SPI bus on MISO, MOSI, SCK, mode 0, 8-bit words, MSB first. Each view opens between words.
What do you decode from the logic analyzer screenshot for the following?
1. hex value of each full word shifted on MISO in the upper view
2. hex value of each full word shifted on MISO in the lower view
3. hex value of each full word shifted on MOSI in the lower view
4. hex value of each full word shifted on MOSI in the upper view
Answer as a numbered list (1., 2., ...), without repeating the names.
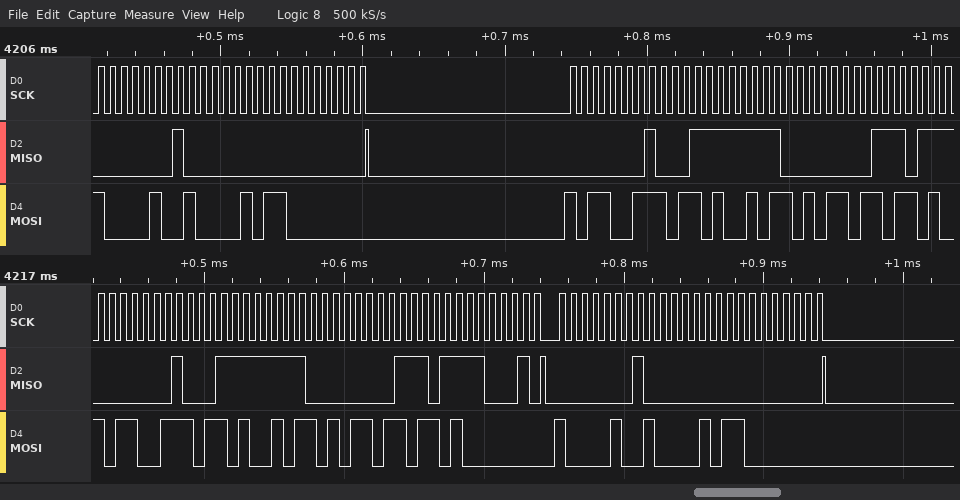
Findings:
1. 01, 00, 00, 01, 1F, E0, 1D
2. 01, 1F, E0, 1D, E2, 01, 00, 00
3. B3, B4, B5, B6, 80, 84, 85, 80
4. 84, 85, 80, B3, B4, B5, B6
